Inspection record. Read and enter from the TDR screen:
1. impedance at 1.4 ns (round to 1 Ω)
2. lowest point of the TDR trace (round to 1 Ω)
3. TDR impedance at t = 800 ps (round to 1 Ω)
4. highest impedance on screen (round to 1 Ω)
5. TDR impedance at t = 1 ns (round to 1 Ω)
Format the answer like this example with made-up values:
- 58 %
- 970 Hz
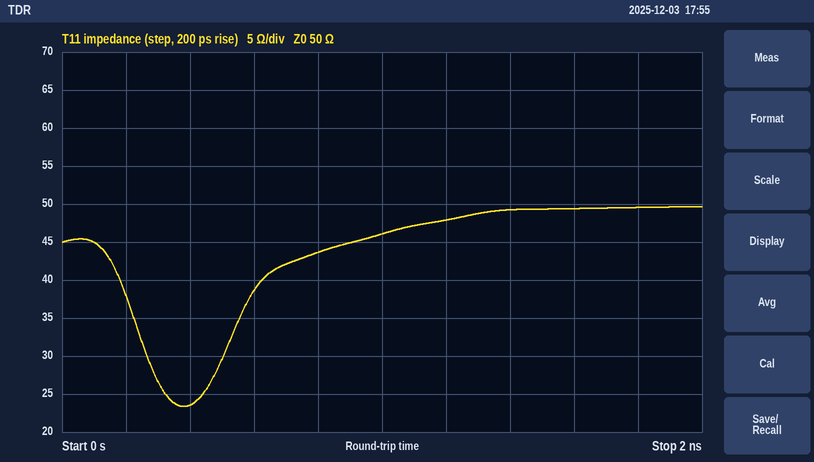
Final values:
- 49 Ω
- 23 Ω
- 44 Ω
- 50 Ω
- 46 Ω
